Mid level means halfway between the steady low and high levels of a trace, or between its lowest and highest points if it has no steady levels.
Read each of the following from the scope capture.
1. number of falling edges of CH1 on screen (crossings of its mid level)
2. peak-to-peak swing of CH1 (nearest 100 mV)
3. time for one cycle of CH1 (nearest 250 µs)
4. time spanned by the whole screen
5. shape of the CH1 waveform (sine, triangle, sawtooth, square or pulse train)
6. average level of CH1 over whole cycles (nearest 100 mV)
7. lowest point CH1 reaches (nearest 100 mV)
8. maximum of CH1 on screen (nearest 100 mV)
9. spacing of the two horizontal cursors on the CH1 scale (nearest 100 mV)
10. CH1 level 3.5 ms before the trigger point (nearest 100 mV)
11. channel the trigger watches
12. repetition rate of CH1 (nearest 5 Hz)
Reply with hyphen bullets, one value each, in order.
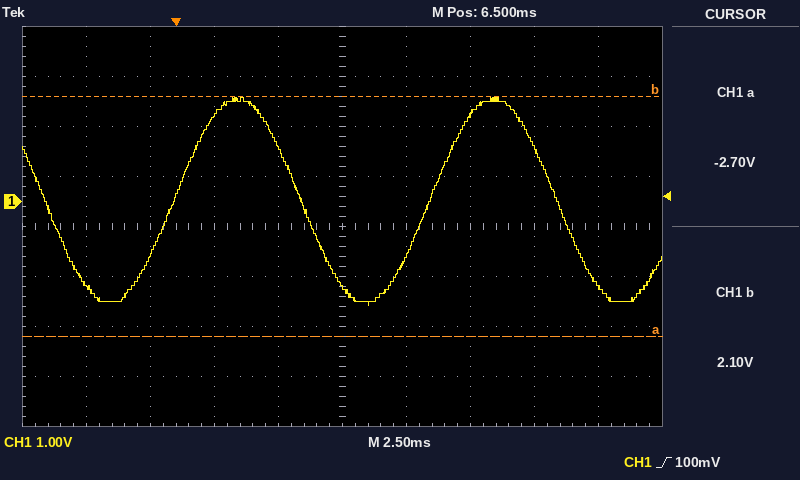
- 3
- 4.2 V
- 10.00 ms
- 25 ms
- sine
- 0.0 V
- -2.1 V
- 2.1 V
- 4.8 V
- -1.7 V
- CH1
- 100 Hz
